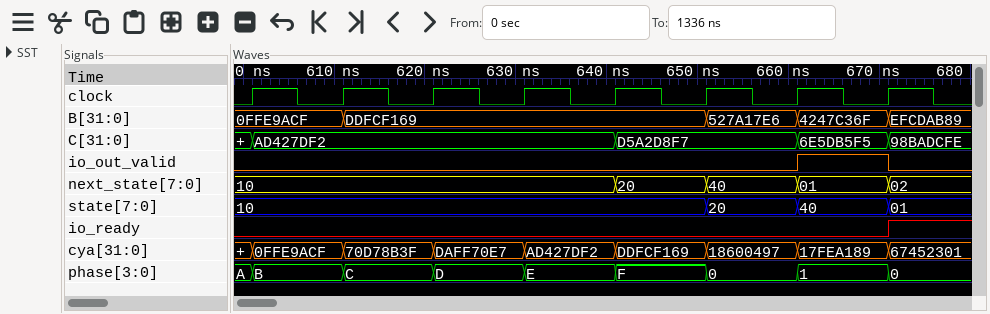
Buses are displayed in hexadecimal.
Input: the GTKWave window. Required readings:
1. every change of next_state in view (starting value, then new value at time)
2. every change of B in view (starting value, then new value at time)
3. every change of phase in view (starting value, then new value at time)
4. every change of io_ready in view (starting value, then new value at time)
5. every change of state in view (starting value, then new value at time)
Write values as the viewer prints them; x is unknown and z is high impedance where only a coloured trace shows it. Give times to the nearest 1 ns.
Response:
10, 20 at 641 ns, 40 at 651 ns, 01 at 661 ns, 02 at 671 ns
0FFE9ACF, DDFCF169 at 611 ns, 527A17E6 at 651 ns, 4247C36F at 661 ns, EFCDAB89 at 671 ns
A, B at 601 ns, C at 611 ns, D at 621 ns, E at 631 ns, F at 641 ns, 0 at 651 ns, 1 at 661 ns, 0 at 671 ns
0, 1 at 671 ns
10, 20 at 651 ns, 40 at 661 ns, 01 at 671 ns
